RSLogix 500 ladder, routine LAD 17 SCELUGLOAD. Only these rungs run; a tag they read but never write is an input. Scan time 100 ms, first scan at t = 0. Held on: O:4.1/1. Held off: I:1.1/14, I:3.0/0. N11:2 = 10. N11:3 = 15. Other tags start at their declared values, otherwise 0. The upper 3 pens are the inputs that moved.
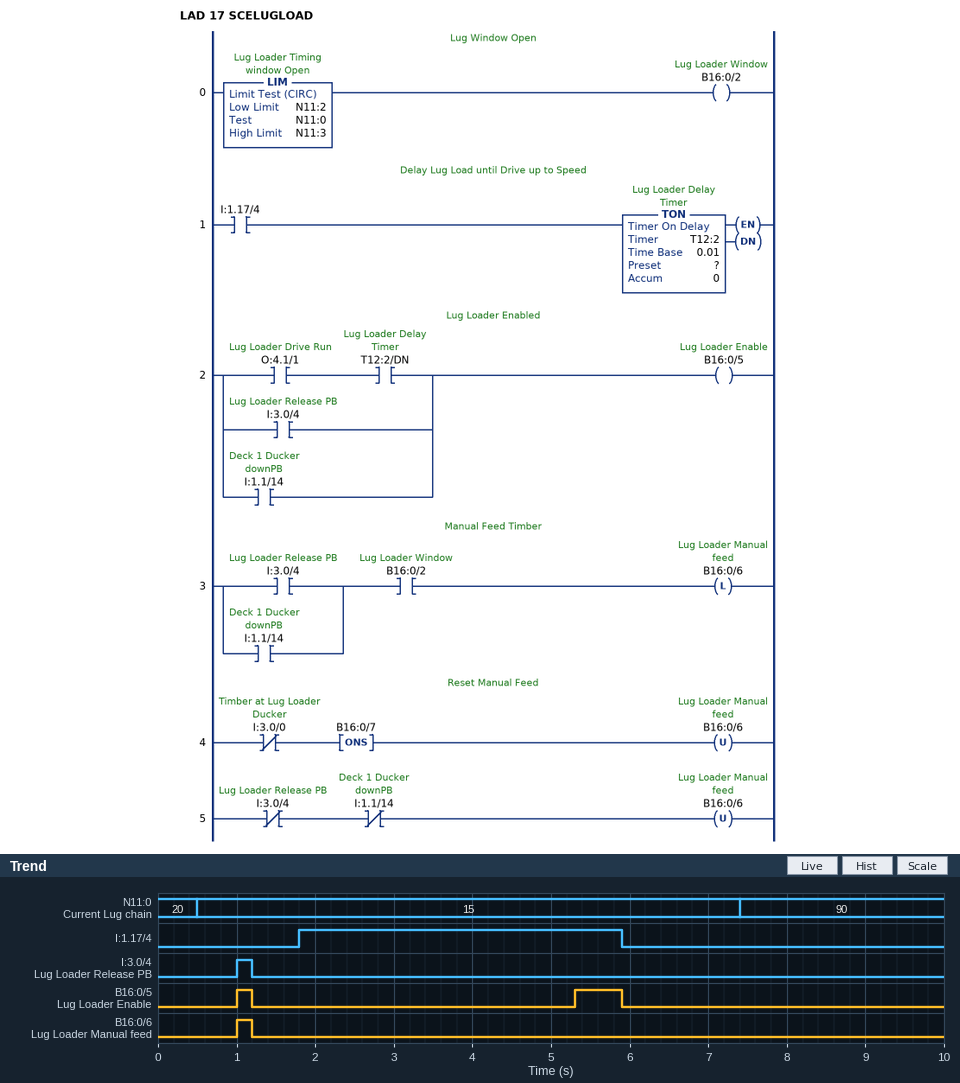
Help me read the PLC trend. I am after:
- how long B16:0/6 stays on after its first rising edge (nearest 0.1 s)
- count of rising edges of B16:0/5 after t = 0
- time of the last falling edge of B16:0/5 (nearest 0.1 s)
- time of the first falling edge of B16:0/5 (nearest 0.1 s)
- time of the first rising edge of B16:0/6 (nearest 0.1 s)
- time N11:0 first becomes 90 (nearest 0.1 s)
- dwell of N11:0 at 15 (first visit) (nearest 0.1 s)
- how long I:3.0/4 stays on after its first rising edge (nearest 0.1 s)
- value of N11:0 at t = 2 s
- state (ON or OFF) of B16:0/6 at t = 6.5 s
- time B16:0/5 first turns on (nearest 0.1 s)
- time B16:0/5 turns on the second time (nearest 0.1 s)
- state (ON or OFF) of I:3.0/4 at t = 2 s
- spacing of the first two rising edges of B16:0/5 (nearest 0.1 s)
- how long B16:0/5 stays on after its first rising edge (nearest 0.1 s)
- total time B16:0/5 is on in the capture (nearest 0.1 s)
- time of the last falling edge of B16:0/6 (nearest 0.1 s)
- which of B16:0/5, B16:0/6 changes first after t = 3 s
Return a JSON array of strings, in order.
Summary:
["0.2 s", "2", "5.9 s", "1.2 s", "1.0 s", "7.4 s", "6.9 s", "0.2 s", "15", "OFF", "1.0 s", "5.3 s", "OFF", "4.3 s", "0.2 s", "0.8 s", "1.2 s", "B16:0/5"]
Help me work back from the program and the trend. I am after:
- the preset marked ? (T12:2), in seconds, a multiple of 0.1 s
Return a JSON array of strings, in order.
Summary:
["3.5 s"]
